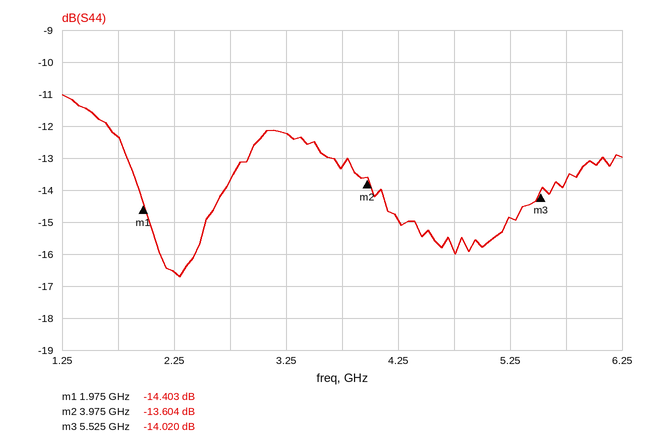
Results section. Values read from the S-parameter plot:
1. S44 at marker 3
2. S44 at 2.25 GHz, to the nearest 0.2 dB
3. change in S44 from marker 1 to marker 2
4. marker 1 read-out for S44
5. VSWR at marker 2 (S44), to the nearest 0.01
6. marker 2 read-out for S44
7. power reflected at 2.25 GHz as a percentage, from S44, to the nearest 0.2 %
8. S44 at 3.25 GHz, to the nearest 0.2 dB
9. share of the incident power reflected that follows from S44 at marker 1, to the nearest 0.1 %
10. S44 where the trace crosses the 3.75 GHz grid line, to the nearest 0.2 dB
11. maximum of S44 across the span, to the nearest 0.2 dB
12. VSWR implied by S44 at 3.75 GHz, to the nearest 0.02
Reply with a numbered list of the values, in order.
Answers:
1. -14.020 dB
2. -16.6 dB
3. 0.799 dB
4. -14.403 dB
5. 1.53
6. -13.604 dB
7. 2.2 %
8. -12.2 dB
9. 3.6 %
10. -13.2 dB
11. -11.0 dB
12. 1.56
